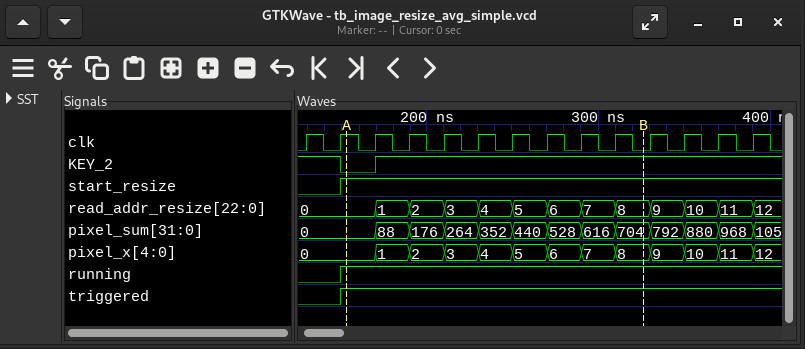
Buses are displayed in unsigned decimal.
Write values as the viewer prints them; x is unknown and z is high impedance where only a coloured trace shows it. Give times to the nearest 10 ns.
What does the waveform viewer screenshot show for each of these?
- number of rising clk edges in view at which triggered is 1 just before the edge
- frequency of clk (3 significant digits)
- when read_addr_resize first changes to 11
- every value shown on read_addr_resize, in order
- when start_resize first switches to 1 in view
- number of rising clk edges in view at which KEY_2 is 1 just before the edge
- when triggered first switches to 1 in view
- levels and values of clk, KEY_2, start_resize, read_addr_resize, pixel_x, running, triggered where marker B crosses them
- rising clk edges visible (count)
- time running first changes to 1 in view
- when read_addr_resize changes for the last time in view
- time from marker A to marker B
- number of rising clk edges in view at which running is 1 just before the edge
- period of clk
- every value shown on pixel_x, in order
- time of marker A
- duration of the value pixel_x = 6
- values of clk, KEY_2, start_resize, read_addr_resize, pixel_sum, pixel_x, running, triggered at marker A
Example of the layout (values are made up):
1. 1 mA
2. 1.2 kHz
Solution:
1. 12
2. 50.0 MHz
3. 370 ns
4. 0, 1, 2, 3, 4, 5, 6, 7, 8, 9, 10, 11, 12
5. 150 ns
6. 13
7. 150 ns
8. clk=0, KEY_2=1, start_resize=1, read_addr_resize=8, pixel_x=8, running=1, triggered=1
9. 14
10. 150 ns
11. 390 ns
12. 170 ns
13. 12
14. 20 ns
15. 0, 1, 2, 3, 4, 5, 6, 7, 8, 9, 10, 11, 12
16. 150 ns
17. 20 ns
18. clk=1, KEY_2=0, start_resize=1, read_addr_resize=0, pixel_sum=0, pixel_x=0, running=1, triggered=1
